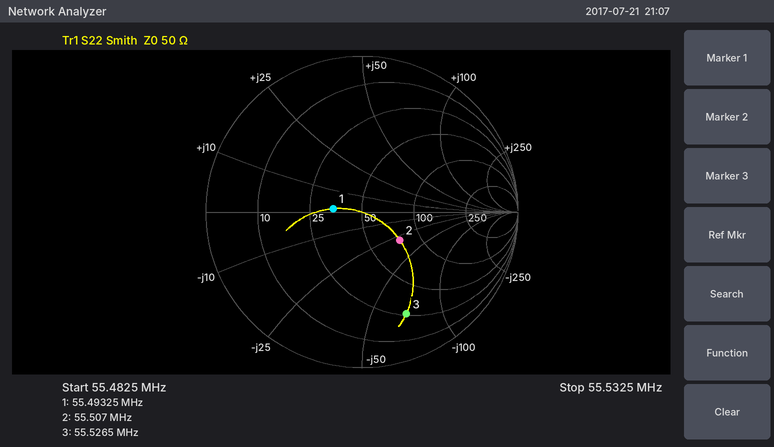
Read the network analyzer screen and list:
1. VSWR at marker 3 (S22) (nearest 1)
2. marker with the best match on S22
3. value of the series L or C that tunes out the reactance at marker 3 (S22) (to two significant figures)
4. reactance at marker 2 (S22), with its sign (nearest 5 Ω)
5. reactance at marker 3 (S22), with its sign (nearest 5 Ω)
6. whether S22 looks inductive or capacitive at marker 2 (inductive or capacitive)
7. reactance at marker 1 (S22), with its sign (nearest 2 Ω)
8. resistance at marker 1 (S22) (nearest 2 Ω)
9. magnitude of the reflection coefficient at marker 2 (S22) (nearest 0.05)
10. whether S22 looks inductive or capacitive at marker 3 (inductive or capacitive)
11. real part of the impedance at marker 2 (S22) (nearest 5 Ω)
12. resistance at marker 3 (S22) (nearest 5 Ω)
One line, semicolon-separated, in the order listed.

6; marker 1; 200 nH; -30 Ω; -70 Ω; capacitive; +2 Ω; 34 Ω; 0.30; capacitive; 75 Ω; 25 Ω
